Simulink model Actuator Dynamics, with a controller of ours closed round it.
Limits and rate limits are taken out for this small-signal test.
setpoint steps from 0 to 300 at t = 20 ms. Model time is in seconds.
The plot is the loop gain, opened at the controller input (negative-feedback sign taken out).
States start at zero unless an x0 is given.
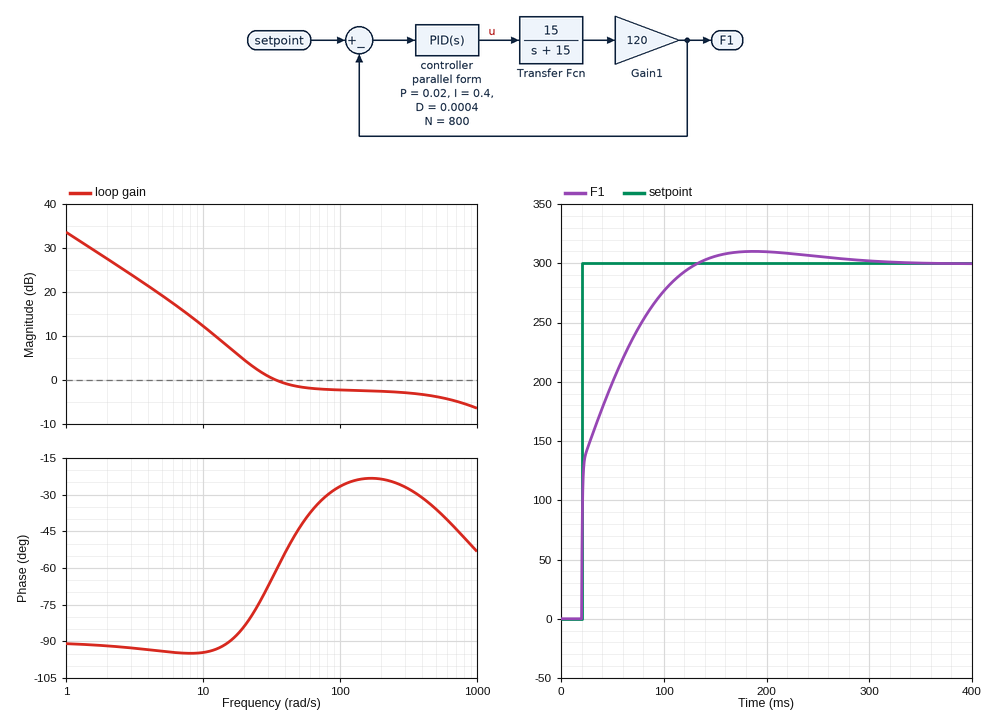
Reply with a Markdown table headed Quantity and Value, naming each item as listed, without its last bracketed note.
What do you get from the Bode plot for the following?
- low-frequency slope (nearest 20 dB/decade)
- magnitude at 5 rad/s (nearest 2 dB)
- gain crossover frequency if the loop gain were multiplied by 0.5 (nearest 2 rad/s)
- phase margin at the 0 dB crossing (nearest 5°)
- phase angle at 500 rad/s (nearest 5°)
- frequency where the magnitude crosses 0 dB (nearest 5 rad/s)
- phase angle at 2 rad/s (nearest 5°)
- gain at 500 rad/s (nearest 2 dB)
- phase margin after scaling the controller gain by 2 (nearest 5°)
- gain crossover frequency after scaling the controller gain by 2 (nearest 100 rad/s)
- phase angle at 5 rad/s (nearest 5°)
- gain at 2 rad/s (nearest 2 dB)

| Quantity | Value |
|---|---|
| low-frequency slope | -20 dB/decade |
| magnitude at 5 rad/s | 20 dB |
| gain crossover frequency if the loop gain were multiplied by 0.5 | 18 rad/s |
| phase margin at the 0 dB crossing | 120° |
| phase angle at 500 rad/s | -35° |
| frequency where the magnitude crosses 0 dB | 35 rad/s |
| phase angle at 2 rad/s | -90° |
| gain at 500 rad/s | -4 dB |
| phase margin after scaling the controller gain by 2 | 130° |
| gain crossover frequency after scaling the controller gain by 2 | 900 rad/s |
| phase angle at 5 rad/s | -95° |
| gain at 2 rad/s | 28 dB |
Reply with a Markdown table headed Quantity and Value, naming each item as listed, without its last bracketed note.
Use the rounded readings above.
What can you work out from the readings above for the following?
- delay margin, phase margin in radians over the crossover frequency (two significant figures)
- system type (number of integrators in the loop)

| Quantity | Value |
|---|---|
| delay margin, phase margin in radians over the crossover frequency | 0.060 s |
| system type | 1 |
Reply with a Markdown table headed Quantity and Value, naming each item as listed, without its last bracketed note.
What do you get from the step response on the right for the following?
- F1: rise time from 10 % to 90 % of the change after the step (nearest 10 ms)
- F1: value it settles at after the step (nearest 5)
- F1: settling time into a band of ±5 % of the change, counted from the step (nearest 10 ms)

| Quantity | Value |
|---|---|
| F1: rise time from 10 % to 90 % of the change after the step | 70 ms |
| F1: value it settles at after the step | 300 |
| F1: settling time into a band of ±5 % of the change, counted from the step | 90 ms |
